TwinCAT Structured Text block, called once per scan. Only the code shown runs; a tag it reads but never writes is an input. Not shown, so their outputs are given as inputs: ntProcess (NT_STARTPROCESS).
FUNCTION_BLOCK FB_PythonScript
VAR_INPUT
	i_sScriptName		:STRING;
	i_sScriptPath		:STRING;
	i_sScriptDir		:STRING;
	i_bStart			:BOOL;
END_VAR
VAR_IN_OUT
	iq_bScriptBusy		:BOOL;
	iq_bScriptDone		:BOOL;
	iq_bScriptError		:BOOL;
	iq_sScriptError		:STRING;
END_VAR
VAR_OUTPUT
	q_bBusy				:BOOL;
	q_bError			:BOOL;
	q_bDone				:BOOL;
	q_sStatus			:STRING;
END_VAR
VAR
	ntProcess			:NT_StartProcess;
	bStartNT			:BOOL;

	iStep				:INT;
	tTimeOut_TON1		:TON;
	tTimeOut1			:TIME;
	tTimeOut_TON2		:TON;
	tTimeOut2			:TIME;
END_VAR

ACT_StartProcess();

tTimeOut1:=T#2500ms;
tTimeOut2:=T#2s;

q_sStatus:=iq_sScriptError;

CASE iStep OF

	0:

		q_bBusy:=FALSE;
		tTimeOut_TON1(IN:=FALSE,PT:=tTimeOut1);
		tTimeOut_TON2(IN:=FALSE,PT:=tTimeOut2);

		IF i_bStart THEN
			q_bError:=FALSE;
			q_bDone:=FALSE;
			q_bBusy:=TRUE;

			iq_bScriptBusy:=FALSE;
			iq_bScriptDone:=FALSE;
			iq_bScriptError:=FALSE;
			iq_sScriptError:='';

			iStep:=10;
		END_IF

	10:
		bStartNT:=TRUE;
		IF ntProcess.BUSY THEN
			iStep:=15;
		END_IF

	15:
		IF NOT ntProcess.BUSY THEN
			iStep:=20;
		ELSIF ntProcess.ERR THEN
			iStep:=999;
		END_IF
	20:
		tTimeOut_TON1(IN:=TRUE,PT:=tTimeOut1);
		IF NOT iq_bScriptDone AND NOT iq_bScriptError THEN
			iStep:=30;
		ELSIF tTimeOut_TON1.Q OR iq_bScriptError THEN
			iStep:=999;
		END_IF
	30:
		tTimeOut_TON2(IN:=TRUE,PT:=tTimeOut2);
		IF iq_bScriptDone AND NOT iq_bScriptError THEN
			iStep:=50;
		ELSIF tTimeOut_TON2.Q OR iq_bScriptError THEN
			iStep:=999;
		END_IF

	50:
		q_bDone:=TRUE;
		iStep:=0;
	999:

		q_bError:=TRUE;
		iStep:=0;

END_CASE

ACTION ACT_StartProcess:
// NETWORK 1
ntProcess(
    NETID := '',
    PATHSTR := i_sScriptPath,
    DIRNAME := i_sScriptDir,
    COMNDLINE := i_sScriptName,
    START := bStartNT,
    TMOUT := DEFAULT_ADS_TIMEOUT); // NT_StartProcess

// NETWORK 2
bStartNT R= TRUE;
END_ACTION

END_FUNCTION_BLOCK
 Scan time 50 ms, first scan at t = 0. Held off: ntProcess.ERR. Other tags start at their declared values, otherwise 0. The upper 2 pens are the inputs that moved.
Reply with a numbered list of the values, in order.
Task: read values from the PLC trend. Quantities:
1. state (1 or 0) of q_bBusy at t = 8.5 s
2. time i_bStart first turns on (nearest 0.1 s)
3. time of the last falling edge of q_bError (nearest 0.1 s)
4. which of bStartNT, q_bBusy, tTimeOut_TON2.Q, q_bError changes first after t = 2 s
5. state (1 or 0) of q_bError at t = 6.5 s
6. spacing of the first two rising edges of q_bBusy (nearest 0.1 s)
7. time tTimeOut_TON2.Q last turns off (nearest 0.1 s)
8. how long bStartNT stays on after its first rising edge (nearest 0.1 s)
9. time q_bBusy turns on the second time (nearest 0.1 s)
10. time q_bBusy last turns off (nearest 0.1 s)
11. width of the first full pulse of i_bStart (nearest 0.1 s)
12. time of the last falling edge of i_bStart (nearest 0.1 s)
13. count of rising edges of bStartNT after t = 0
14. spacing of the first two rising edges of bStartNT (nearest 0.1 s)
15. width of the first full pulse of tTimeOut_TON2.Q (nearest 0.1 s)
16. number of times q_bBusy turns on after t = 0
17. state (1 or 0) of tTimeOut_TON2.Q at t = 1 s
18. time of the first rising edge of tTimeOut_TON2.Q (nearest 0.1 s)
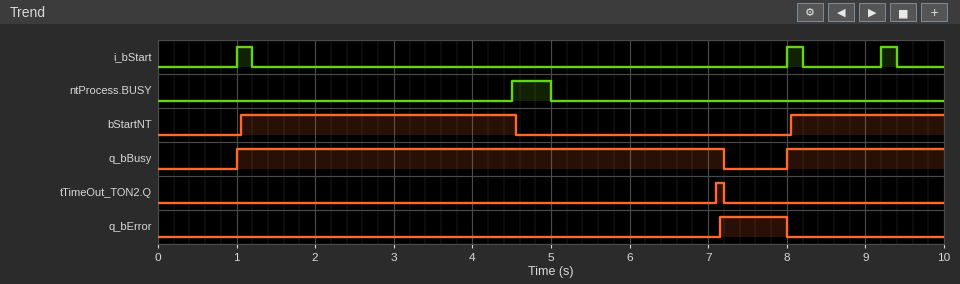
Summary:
1. 1
2. 1.0 s
3. 8.0 s
4. bStartNT
5. 0
6. 7.0 s
7. 7.2 s
8. 3.5 s
9. 8.0 s
10. 7.2 s
11. 0.2 s
12. 9.4 s
13. 2
14. 7.0 s
15. 0.1 s
16. 2
17. 0
18. 7.1 s
